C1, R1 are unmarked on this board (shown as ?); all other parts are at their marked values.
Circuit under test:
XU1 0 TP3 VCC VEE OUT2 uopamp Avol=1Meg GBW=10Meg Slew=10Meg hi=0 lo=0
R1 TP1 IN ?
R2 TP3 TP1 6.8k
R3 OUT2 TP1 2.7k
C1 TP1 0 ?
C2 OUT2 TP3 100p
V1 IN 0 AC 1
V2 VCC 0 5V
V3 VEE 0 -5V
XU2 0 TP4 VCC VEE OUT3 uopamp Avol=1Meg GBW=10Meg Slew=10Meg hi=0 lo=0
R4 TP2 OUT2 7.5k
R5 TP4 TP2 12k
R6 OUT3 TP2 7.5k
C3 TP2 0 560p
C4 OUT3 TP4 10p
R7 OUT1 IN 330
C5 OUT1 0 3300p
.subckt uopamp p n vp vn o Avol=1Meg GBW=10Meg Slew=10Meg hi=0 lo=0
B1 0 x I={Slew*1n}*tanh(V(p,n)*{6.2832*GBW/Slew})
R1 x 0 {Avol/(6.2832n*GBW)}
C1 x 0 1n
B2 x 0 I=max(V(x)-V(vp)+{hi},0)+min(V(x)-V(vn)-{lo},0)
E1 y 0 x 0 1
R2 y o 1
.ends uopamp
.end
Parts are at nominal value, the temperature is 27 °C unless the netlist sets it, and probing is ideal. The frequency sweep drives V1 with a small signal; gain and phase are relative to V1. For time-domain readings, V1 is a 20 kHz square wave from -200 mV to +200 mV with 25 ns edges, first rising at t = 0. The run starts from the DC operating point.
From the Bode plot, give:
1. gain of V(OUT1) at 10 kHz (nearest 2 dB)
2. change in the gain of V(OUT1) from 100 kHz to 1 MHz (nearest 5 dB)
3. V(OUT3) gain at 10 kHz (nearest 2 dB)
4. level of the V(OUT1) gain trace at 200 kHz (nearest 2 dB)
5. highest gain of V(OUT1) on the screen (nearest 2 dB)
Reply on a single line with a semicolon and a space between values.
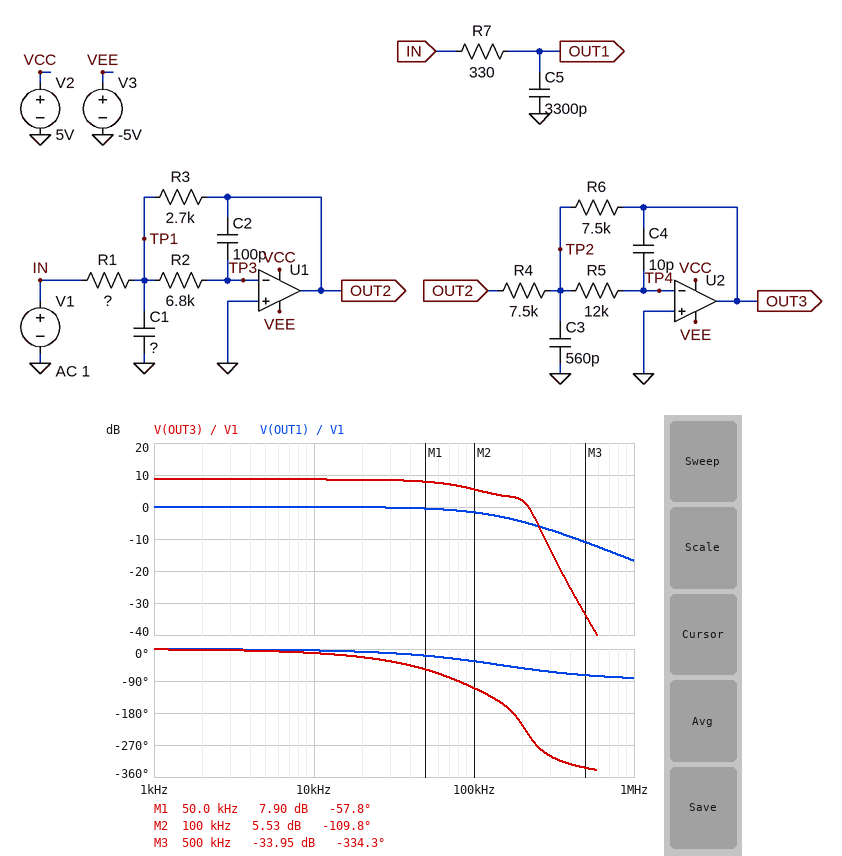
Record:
0 dB; -15 dB; 8 dB; -4 dB; 0 dB
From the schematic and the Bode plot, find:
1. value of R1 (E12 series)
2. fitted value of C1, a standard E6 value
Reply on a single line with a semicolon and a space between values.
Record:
1 kΩ; 1.5 nF
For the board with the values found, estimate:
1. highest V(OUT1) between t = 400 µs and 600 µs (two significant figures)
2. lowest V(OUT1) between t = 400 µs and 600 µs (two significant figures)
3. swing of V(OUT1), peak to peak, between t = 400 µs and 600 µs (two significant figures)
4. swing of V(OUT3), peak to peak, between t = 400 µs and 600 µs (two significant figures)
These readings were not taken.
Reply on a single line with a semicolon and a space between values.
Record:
200 mV; -200 mV; 400 mV; 1.1 V
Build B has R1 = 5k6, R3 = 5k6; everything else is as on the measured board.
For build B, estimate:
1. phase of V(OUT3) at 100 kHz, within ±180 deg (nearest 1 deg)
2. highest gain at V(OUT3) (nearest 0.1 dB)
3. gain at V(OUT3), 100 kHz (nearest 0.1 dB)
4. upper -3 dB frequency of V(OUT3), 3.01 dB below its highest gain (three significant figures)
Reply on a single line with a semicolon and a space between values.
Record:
-153 deg; 3.2 dB; -3.1 dB; 81.4 kHz
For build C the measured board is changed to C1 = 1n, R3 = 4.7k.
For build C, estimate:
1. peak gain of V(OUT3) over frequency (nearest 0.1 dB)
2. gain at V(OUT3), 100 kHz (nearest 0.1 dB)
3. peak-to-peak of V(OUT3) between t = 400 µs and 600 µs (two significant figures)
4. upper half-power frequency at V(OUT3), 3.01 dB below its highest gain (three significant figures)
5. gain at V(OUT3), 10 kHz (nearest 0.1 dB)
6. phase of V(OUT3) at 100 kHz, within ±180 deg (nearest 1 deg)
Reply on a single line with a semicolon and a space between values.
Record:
13.4 dB; 6.4 dB; 1.9 V; 46.5 kHz; 13.2 dB; -112 deg
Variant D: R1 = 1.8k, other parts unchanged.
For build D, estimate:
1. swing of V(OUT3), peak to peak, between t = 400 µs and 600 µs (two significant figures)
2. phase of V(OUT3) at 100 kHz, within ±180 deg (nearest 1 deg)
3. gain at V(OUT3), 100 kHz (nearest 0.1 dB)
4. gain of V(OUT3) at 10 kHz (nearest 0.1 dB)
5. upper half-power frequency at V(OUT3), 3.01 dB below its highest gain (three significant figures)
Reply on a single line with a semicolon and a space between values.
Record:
770 mV; -111 deg; 3.4 dB; 3.6 dB; 131 kHz
